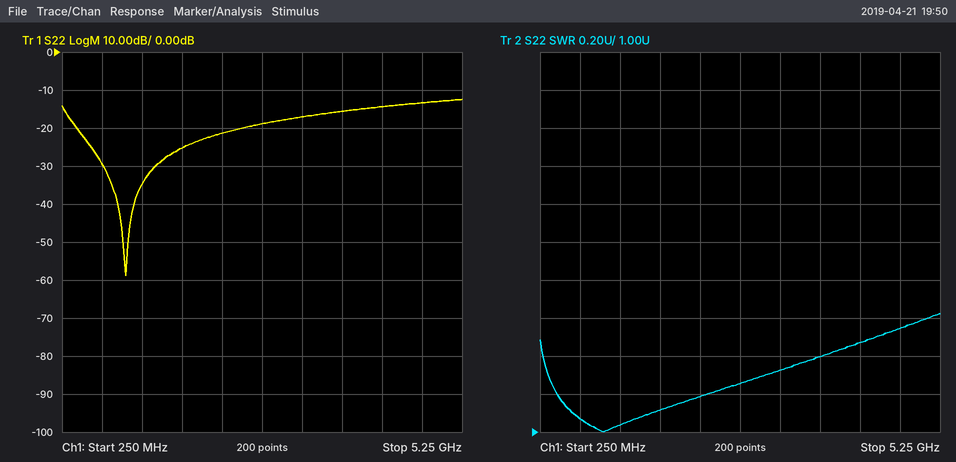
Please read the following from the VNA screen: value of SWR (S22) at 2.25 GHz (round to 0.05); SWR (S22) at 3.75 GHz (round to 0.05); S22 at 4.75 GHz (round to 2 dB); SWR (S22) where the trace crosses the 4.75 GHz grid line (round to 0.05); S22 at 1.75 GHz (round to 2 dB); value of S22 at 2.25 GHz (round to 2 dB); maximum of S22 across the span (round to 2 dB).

1.20
1.40
-14 dB
1.55
-26 dB
-22 dB
-12 dB
